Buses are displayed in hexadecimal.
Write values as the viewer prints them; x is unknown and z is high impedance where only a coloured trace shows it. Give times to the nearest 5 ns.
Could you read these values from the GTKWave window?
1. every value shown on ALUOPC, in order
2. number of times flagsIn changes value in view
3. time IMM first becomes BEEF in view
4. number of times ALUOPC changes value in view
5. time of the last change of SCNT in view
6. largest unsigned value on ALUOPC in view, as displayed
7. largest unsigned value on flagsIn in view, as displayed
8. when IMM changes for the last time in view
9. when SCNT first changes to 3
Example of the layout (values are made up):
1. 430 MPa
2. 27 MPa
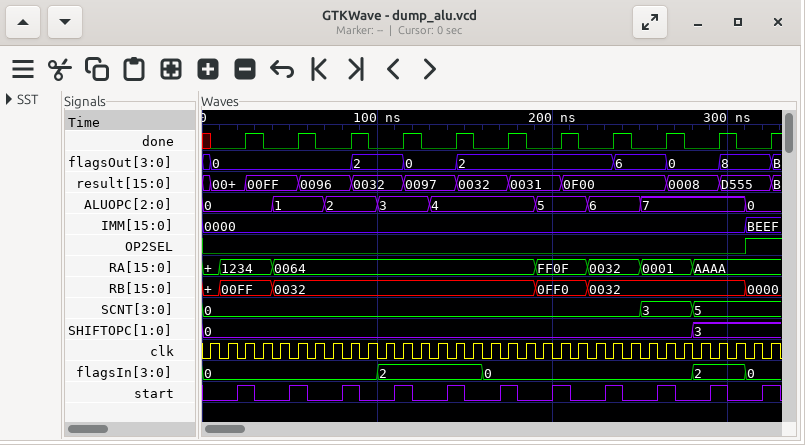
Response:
1. 0, 1, 2, 3, 4, 5, 6, 7, 0
2. 4
3. 310 ns
4. 8
5. 280 ns
6. 7
7. 2
8. 310 ns
9. 250 ns
